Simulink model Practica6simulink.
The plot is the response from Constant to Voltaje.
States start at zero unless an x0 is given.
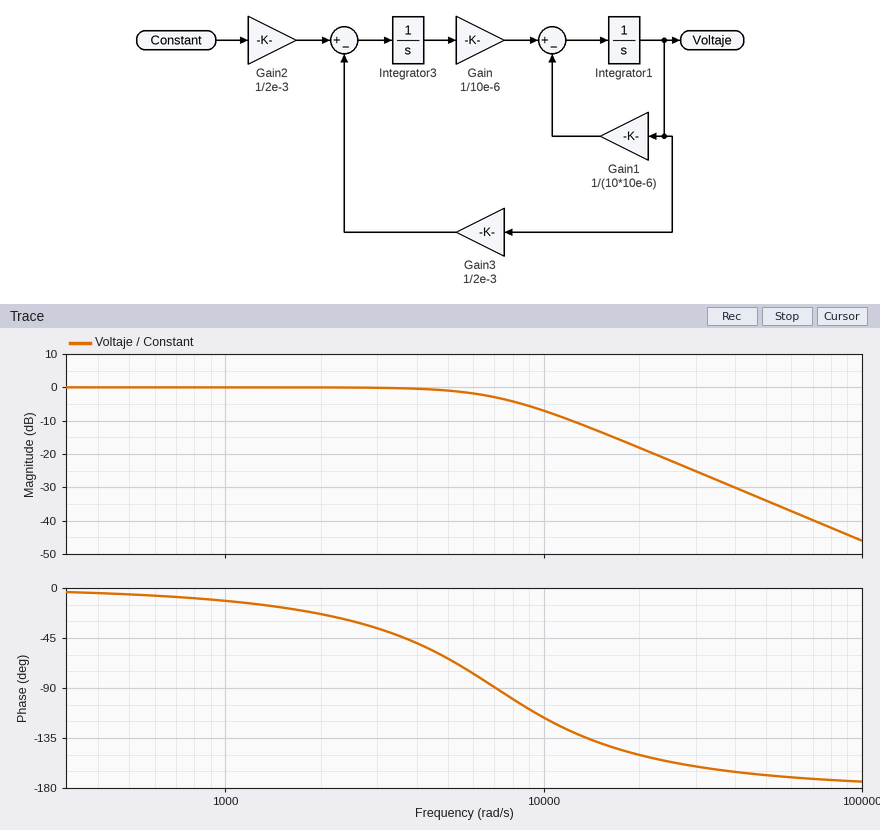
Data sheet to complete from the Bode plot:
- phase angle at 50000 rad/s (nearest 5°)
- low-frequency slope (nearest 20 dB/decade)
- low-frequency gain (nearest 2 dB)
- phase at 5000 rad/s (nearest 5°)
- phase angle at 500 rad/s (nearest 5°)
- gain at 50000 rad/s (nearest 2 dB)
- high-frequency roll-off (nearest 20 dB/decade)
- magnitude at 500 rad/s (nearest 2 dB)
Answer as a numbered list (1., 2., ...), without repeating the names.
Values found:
1. -170°
2. 0 dB/decade
3. 0 dB
4. -65°
5. -5°
6. -34 dB
7. -40 dB/decade
8. 0 dB
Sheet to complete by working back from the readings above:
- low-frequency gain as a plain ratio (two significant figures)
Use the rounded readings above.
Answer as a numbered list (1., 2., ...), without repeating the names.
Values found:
1. 1.0
